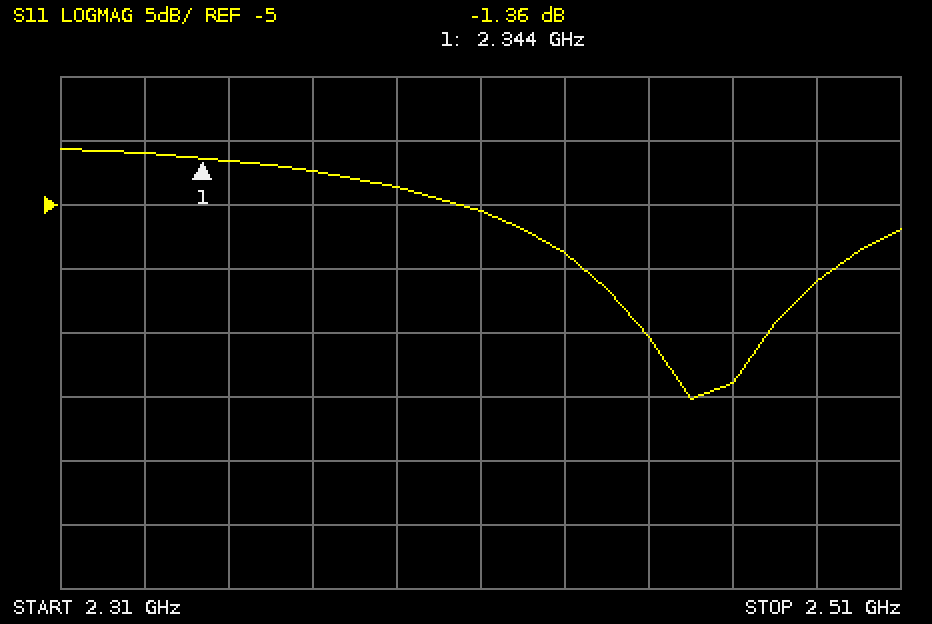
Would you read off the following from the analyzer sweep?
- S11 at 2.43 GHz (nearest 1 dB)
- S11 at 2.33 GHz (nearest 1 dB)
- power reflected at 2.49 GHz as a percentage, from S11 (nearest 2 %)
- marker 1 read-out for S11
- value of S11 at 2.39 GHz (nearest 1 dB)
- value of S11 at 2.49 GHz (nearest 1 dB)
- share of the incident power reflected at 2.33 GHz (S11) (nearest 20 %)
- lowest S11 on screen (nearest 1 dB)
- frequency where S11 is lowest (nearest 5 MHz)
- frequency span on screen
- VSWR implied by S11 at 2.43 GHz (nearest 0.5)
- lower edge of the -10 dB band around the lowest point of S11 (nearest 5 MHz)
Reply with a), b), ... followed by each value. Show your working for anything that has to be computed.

a) -9 dB
b) -1 dB
c) 10^(-11/10) ≈ 8 %
d) -1.36 dB
e) -4 dB
f) -11 dB
g) 10^(-1/10) ≈ 79.4 %, so 80 % to the nearest 20 %
h) -20 dB
i) 2.460 GHz
j) 200 MHz
k) |Γ| = 10^(-9/20) = 0.3548; VSWR = (1 + 0.3548)/(1 − 0.3548) ≈ 2.10, so 2.0 to the nearest 0.5
l) 2.435 GHz
